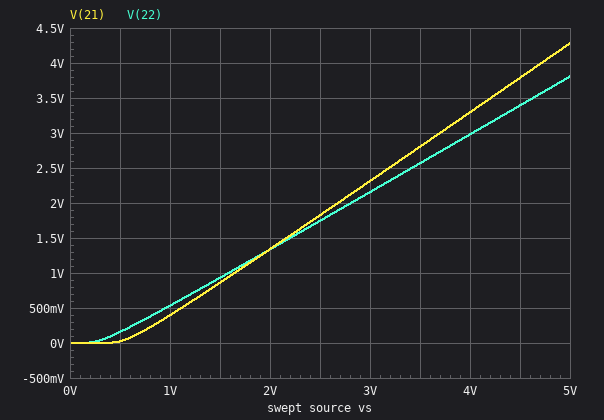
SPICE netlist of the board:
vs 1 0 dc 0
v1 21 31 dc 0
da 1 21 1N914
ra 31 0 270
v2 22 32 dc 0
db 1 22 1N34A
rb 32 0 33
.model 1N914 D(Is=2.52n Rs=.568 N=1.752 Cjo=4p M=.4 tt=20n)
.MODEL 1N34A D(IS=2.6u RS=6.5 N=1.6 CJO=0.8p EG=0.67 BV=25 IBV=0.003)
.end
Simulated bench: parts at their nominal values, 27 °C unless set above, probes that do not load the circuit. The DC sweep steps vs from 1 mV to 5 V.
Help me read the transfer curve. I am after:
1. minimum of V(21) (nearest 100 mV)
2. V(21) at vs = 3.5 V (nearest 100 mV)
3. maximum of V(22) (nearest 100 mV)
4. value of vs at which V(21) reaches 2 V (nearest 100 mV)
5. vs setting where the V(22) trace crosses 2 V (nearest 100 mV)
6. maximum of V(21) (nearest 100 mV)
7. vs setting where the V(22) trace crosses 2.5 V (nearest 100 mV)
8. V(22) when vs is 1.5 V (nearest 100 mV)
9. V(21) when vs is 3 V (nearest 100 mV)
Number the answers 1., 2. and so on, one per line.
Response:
1. 0 V
2. 2.8 V
3. 3.8 V
4. 2.7 V
5. 2.8 V
6. 4.3 V
7. 3.4 V
8. 900 mV
9. 2.3 V
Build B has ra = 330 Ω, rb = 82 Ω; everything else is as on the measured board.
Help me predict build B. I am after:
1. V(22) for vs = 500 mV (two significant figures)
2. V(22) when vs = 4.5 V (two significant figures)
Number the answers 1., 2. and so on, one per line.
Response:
1. 200 mV
2. 3.8 V
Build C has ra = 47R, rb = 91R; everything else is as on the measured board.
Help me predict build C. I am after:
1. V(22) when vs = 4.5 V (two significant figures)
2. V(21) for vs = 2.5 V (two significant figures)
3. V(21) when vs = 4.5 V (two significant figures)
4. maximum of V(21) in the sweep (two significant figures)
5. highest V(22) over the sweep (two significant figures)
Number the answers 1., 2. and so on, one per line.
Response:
1. 3.8 V
2. 1.7 V
3. 3.7 V
4. 4.2 V
5. 4.3 V
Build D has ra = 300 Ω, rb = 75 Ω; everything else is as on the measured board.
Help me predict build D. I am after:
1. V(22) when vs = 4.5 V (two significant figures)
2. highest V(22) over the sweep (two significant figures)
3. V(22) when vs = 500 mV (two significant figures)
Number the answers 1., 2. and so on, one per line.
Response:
1. 3.8 V
2. 4.2 V
3. 200 mV
